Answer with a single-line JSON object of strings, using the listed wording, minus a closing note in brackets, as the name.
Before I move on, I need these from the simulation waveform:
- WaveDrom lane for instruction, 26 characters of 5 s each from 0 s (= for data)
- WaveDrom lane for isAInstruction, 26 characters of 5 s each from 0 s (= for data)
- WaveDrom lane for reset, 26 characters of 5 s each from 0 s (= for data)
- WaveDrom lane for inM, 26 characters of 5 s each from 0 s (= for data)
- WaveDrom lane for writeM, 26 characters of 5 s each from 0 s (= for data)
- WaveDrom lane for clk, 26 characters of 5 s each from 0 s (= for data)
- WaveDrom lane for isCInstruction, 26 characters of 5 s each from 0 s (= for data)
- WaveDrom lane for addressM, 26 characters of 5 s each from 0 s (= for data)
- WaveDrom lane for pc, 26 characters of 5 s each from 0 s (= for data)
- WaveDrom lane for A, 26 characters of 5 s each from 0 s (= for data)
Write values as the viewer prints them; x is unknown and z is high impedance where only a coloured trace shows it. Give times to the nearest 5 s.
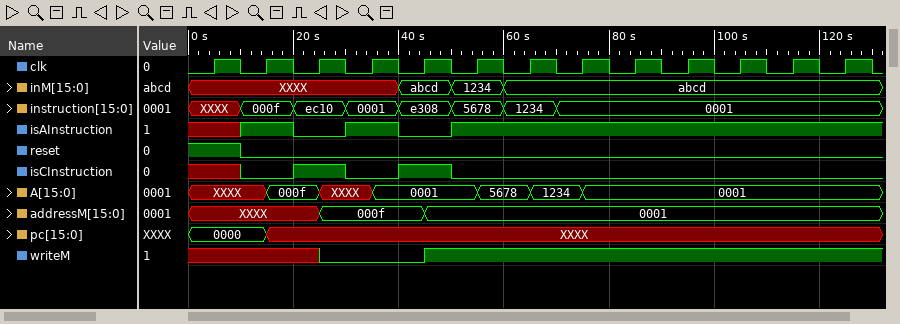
{"WaveDrom lane for instruction, 26 characters of 5 s each from 0 s": "{name: 'instruction', wave: 'x.=.=.=.=.=.=.=...........', data: '000f ec10 0001 e308 5678 1234 0001'}", "WaveDrom lane for isAInstruction, 26 characters of 5 s each from 0 s": "{name: 'isAInstruction', wave: 'x.1.0.1.0.1...............'}", "WaveDrom lane for reset, 26 characters of 5 s each from 0 s": "{name: 'reset', wave: '1.0.......................'}", "WaveDrom lane for inM, 26 characters of 5 s each from 0 s": "{name: 'inM', wave: 'x.......=.=.=.............', data: 'abcd 1234 abcd'}", "WaveDrom lane for writeM, 26 characters of 5 s each from 0 s": "{name: 'writeM', wave: 'x....0...1................'}", "WaveDrom lane for clk, 26 characters of 5 s each from 0 s": "{name: 'clk', wave: '01010101010101010101010101'}", "WaveDrom lane for isCInstruction, 26 characters of 5 s each from 0 s": "{name: 'isCInstruction', wave: 'x.0.1.0.1.0...............'}", "WaveDrom lane for addressM, 26 characters of 5 s each from 0 s": "{name: 'addressM', wave: 'x....=...=................', data: '000f 0001'}", "WaveDrom lane for pc, 26 characters of 5 s each from 0 s": "{name: 'pc', wave: '=..=......................', data: '0000 XXXX'}", "WaveDrom lane for A, 26 characters of 5 s each from 0 s": "{name: 'A', wave: 'x..=.x.=...=.=.=..........', data: '000f 0001 5678 1234 0001'}"}
